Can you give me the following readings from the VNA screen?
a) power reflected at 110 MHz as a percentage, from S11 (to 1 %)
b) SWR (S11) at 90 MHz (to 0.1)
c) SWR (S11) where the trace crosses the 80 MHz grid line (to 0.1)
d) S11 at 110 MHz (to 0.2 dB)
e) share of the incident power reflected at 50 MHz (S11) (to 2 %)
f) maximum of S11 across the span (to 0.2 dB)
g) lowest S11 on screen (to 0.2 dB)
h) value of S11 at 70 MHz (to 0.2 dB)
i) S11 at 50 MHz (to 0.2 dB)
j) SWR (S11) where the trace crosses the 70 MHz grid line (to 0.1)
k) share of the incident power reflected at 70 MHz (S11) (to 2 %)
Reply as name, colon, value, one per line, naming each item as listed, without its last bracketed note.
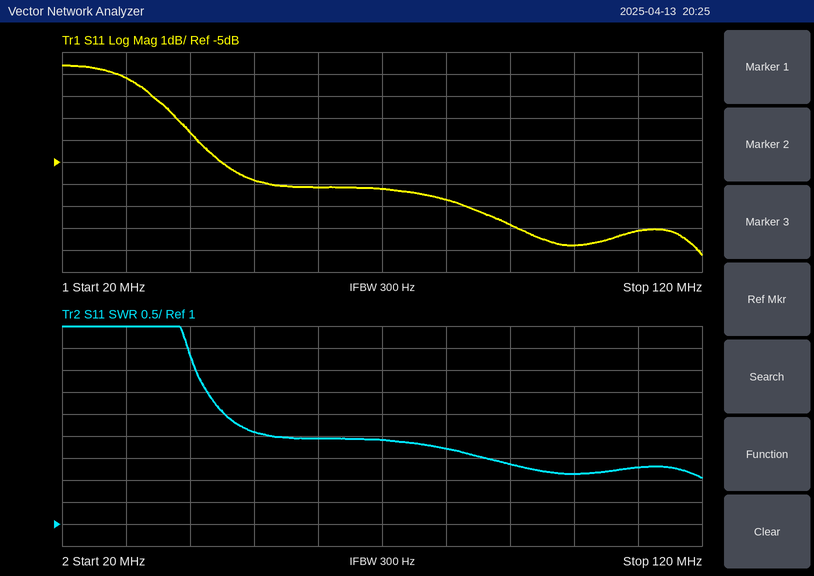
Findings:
power reflected at 110 MHz as a percentage, from S11: 15 %
SWR (S11) at 90 MHz: 2.4
SWR (S11) where the trace crosses the 80 MHz grid line: 2.7
S11 at 110 MHz: -8.2 dB
share of the incident power reflected at 50 MHz (S11): 26 %
maximum of S11 across the span: -0.6 dB
lowest S11 on screen: -9.2 dB
value of S11 at 70 MHz: -6.2 dB
S11 at 50 MHz: -5.8 dB
SWR (S11) where the trace crosses the 70 MHz grid line: 2.9
share of the incident power reflected at 70 MHz (S11): 24 %
